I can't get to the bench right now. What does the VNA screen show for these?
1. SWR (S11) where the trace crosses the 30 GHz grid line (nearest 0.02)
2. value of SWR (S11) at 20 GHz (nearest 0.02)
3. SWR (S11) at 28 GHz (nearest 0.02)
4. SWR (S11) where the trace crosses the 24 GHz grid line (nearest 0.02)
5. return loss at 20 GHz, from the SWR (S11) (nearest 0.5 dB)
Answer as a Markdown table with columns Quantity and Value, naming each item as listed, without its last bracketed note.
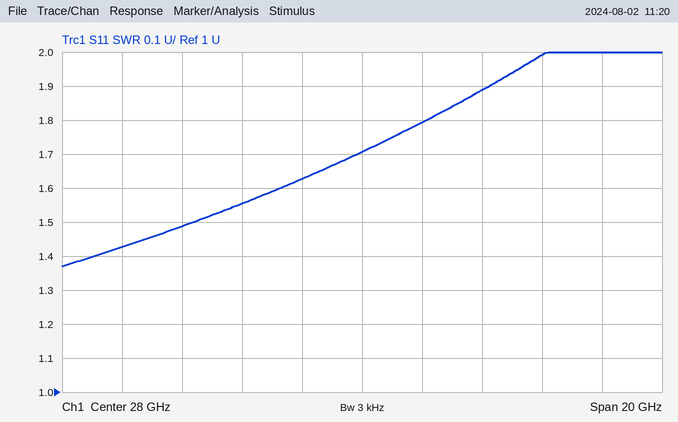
| Quantity | Value |
|---|---|
| SWR (S11) where the trace crosses the 30 GHz grid line | 1.80 |
| value of SWR (S11) at 20 GHz | 1.42 |
| SWR (S11) at 28 GHz | 1.70 |
| SWR (S11) where the trace crosses the 24 GHz grid line | 1.56 |
| return loss at 20 GHz, from the SWR (S11) | 15.0 dB |
